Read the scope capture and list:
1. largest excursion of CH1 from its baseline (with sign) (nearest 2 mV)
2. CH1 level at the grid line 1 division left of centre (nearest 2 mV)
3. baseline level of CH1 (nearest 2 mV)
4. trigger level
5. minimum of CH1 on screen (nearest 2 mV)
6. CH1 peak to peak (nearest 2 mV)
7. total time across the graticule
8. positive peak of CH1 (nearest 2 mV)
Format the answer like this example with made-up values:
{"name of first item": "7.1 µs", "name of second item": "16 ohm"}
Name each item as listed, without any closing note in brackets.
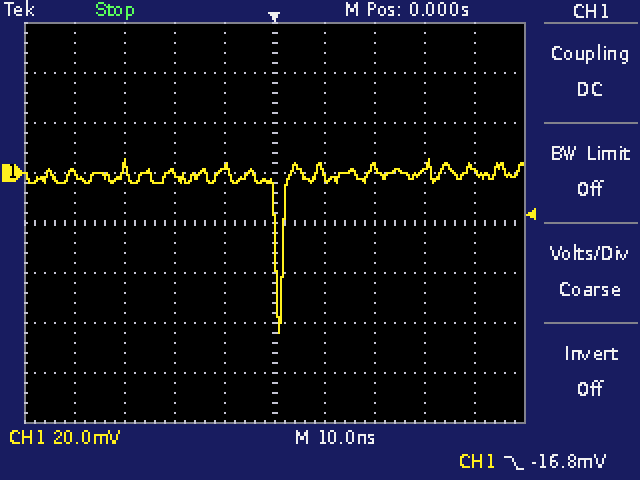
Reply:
{"largest excursion of CH1 from its baseline (with sign)": "-62 mV", "CH1 level at the grid line 1 division left of centre": "2 mV", "baseline level of CH1": "-2 mV", "trigger level": "-16.8 mV", "minimum of CH1 on screen": "-64 mV", "CH1 peak to peak": "70 mV", "total time across the graticule": "100 ns", "positive peak of CH1": "6 mV"}
